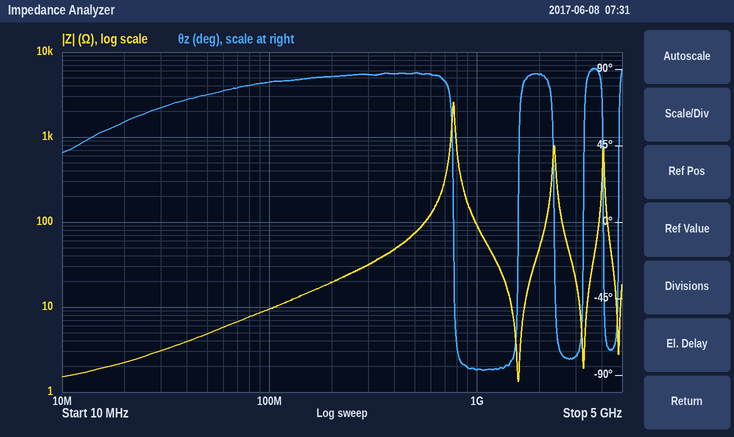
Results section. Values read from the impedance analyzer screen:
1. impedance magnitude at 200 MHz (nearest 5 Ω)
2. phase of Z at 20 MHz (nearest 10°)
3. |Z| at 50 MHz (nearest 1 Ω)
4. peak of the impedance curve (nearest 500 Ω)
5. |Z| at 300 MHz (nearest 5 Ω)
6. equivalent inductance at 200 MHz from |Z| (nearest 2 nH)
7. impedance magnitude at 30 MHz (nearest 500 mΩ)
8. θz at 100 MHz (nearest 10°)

20 Ω
60°
5 Ω
2.5 kΩ
30 Ω
16 nH
3.0 Ω
80°
